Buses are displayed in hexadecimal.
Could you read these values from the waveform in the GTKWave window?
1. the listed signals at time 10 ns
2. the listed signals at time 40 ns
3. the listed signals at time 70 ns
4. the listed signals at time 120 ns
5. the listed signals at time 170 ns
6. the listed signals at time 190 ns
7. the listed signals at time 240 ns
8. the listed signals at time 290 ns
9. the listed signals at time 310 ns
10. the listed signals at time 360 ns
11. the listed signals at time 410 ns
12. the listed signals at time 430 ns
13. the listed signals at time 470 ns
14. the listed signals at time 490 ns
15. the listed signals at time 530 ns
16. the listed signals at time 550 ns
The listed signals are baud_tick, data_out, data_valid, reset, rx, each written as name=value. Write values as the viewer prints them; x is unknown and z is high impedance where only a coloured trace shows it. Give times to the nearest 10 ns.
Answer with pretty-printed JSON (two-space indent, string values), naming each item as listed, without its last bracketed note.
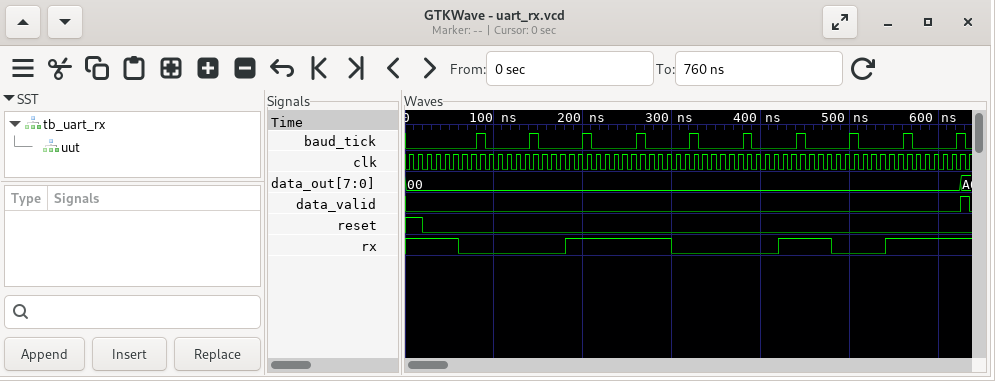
{
  "the listed signals at time 10 ns": "baud_tick=0, data_out=00, data_valid=0, reset=1, rx=1",
  "the listed signals at time 40 ns": "baud_tick=0, data_out=00, data_valid=0, reset=0, rx=1",
  "the listed signals at time 70 ns": "baud_tick=0, data_out=00, data_valid=0, reset=0, rx=0",
  "the listed signals at time 120 ns": "baud_tick=0, data_out=00, data_valid=0, reset=0, rx=0",
  "the listed signals at time 170 ns": "baud_tick=0, data_out=00, data_valid=0, reset=0, rx=0",
  "the listed signals at time 190 ns": "baud_tick=0, data_out=00, data_valid=0, reset=0, rx=1",
  "the listed signals at time 240 ns": "baud_tick=0, data_out=00, data_valid=0, reset=0, rx=1",
  "the listed signals at time 290 ns": "baud_tick=0, data_out=00, data_valid=0, reset=0, rx=1",
  "the listed signals at time 310 ns": "baud_tick=0, data_out=00, data_valid=0, reset=0, rx=0",
  "the listed signals at time 360 ns": "baud_tick=0, data_out=00, data_valid=0, reset=0, rx=0",
  "the listed signals at time 410 ns": "baud_tick=0, data_out=00, data_valid=0, reset=0, rx=0",
  "the listed signals at time 430 ns": "baud_tick=0, data_out=00, data_valid=0, reset=0, rx=1",
  "the listed signals at time 470 ns": "baud_tick=0, data_out=00, data_valid=0, reset=0, rx=1",
  "the listed signals at time 490 ns": "baud_tick=0, data_out=00, data_valid=0, reset=0, rx=0",
  "the listed signals at time 530 ns": "baud_tick=0, data_out=00, data_valid=0, reset=0, rx=0",
  "the listed signals at time 550 ns": "baud_tick=0, data_out=00, data_valid=0, reset=0, rx=1"
}
